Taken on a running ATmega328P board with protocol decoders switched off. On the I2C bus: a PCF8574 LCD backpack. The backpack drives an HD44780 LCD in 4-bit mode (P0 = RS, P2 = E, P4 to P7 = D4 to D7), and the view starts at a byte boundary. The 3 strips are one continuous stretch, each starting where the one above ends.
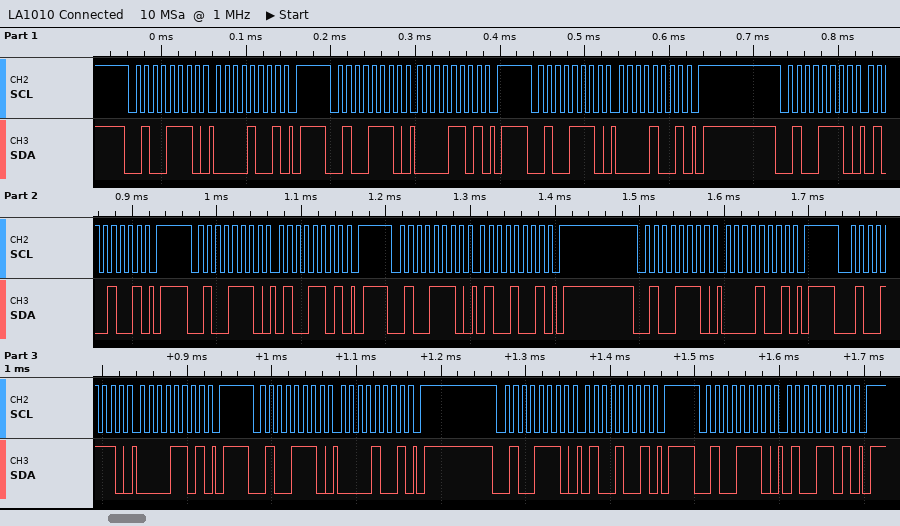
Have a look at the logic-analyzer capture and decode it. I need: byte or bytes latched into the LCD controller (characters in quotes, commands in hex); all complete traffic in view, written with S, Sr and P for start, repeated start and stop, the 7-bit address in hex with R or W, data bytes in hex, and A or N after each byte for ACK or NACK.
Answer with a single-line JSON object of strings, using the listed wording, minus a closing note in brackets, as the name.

{"byte or bytes latched into the LCD controller": "data 0x04", "all complete traffic in view, written with S, Sr and P for start, repeated start and stop, the 7-bit address in hex with R or W, data bytes in hex, and A or N after each byte for ACK or NACK": "S 27W A 09 A P S 27W A 0D A P S 27W A 09 A P S 27W A 49 A P S 27W A 4D A P S 27W A 49 A P S 27W A 09 A P S 27W A 0D A P S 27W A 09 A P S 27W A 49 A P S 27W A 4D A P"}
